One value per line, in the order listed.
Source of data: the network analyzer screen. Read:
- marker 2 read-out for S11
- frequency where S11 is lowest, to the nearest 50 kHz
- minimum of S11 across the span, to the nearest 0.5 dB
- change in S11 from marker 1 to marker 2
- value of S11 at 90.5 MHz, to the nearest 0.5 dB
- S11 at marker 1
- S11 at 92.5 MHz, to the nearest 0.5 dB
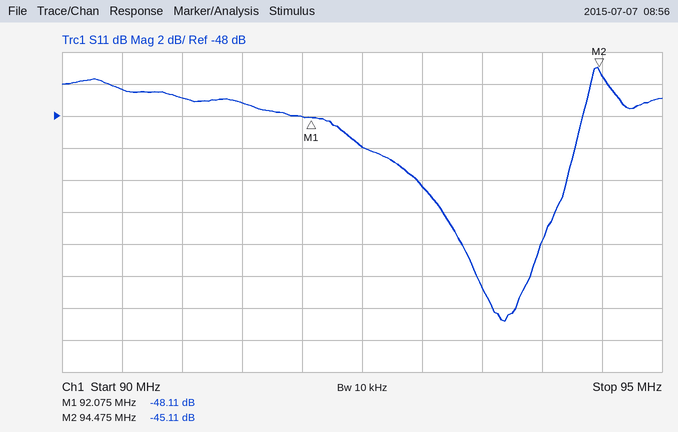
-45.11 dB
93.70 MHz
-61.0 dB
3.00 dB
-46.5 dB
-48.11 dB
-50.0 dB
